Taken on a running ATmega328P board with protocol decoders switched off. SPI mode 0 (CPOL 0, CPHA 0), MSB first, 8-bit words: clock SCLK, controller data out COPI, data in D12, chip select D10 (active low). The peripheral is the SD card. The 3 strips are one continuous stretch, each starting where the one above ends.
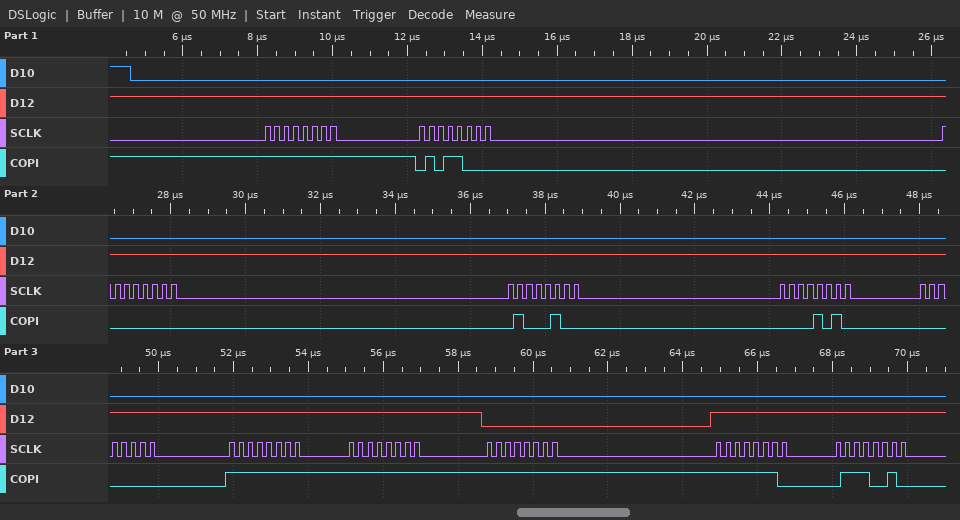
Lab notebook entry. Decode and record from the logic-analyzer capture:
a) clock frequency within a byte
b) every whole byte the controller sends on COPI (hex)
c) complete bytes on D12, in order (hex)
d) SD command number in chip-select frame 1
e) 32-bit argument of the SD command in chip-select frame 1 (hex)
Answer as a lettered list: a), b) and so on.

a) 4 MHz
b) FF 58 00 44 0A 00 FF FF FF FE 72
c) FF FF FF FF FF FF FF FF 00 FF FF
d) CMD24
e) 0x00440A00
